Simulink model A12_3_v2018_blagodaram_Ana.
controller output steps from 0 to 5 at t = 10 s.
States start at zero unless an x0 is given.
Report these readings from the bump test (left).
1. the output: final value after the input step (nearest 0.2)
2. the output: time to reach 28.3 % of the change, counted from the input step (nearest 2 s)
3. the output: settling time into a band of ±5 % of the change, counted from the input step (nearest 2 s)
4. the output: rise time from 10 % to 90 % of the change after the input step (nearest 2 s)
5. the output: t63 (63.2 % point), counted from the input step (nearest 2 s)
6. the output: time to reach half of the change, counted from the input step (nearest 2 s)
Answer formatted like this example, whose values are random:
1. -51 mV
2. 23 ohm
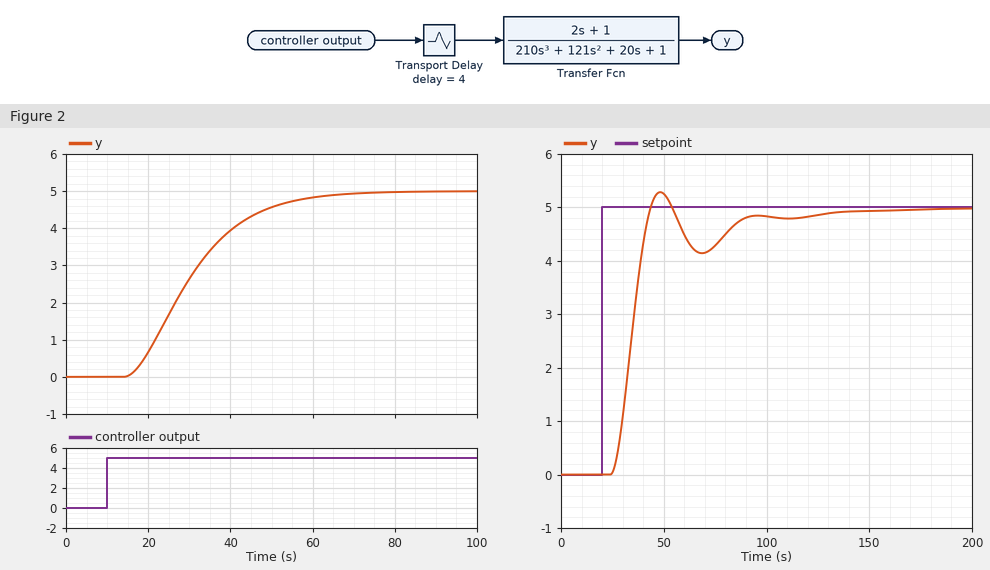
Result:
1. 5.0
2. 14 s
3. 46 s
4. 30 s
5. 24 s
6. 20 s
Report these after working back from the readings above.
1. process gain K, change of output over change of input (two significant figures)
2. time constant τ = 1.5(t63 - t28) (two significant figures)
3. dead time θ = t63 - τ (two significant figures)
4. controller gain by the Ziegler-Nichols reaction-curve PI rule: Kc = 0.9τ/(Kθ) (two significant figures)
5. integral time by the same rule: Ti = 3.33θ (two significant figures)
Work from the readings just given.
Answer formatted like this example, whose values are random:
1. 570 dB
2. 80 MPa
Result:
1. 1.0
2. 15 s
3. 9.0 s
4. 1.5
5. 30 s
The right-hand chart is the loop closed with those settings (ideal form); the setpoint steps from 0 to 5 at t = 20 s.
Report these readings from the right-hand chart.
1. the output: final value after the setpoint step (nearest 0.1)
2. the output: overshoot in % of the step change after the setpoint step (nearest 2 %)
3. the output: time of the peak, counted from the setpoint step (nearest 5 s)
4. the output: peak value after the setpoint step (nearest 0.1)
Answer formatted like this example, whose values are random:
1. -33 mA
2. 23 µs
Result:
1. 5.0
2. 6 %
3. 30 s
4. 5.3
